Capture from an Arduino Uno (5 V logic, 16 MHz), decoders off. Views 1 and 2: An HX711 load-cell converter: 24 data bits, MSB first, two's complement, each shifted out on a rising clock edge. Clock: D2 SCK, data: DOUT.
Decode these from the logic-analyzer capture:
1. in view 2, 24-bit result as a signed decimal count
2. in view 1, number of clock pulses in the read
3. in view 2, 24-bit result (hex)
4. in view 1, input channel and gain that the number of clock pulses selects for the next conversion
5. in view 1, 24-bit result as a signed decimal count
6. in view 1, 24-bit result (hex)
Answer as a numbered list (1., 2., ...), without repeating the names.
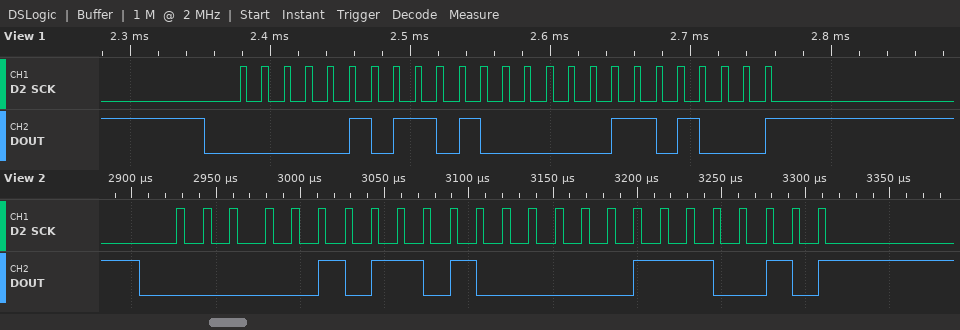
1. 368754
2. 25
3. 0x05A072
4. channel A, gain 128
5. 368744
6. 0x05A068
